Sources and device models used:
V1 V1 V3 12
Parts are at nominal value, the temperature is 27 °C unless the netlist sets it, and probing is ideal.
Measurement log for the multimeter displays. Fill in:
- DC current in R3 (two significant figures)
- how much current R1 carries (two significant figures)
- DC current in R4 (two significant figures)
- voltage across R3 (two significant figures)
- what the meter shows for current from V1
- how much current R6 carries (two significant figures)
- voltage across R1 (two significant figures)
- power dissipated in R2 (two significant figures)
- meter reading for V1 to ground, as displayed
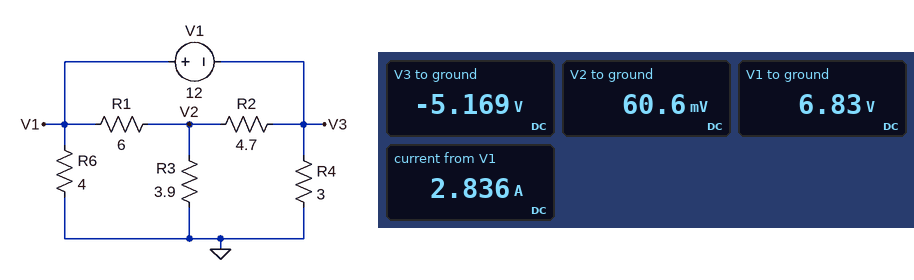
16 mA
1.1 A
1.7 A
61 mV
2.836 A
1.7 A
6.8 V
5.8 W
6.83 V
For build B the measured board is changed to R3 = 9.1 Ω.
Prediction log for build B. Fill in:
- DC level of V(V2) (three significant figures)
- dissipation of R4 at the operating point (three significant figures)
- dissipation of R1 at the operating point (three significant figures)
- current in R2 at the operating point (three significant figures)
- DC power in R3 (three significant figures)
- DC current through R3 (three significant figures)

86.7 mV
8.87 W
7.60 W
1.12 A
826 µW
9.53 mA
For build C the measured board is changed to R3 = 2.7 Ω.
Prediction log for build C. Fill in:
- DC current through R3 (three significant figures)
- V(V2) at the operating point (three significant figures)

18.2 mA
49.1 mV
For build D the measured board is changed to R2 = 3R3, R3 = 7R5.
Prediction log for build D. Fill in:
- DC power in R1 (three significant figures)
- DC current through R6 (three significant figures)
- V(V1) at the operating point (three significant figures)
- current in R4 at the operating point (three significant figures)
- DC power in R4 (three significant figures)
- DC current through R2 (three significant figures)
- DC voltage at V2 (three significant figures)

9.57 W
1.75 A
6.99 V
1.67 A
8.36 W
1.34 A
-585 mV
